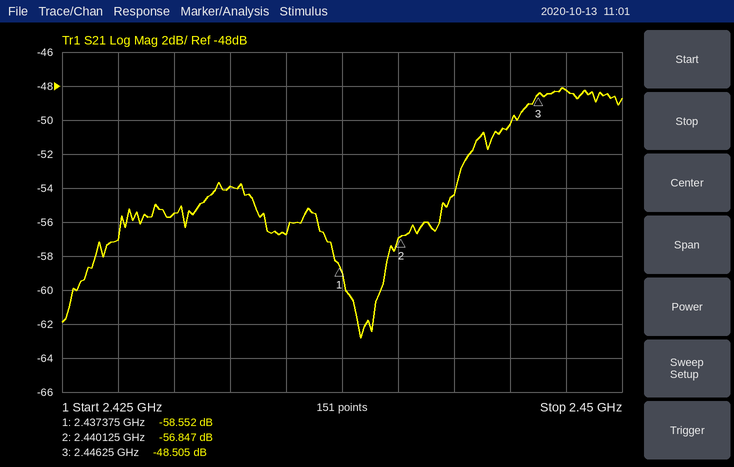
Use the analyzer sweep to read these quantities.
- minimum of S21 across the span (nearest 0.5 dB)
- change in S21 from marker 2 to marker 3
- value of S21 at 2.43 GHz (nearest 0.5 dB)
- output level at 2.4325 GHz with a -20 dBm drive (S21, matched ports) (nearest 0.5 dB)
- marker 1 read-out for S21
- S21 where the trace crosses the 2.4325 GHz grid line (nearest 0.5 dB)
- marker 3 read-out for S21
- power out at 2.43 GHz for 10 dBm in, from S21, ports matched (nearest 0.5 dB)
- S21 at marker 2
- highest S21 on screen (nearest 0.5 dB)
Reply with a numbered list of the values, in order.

1. -63.0 dB
2. 8.342 dB
3. -55.5 dB
4. -74.0 dBm
5. -58.552 dB
6. -54.0 dB
7. -48.505 dB
8. -45.5 dBm
9. -56.847 dB
10. -48.0 dB
